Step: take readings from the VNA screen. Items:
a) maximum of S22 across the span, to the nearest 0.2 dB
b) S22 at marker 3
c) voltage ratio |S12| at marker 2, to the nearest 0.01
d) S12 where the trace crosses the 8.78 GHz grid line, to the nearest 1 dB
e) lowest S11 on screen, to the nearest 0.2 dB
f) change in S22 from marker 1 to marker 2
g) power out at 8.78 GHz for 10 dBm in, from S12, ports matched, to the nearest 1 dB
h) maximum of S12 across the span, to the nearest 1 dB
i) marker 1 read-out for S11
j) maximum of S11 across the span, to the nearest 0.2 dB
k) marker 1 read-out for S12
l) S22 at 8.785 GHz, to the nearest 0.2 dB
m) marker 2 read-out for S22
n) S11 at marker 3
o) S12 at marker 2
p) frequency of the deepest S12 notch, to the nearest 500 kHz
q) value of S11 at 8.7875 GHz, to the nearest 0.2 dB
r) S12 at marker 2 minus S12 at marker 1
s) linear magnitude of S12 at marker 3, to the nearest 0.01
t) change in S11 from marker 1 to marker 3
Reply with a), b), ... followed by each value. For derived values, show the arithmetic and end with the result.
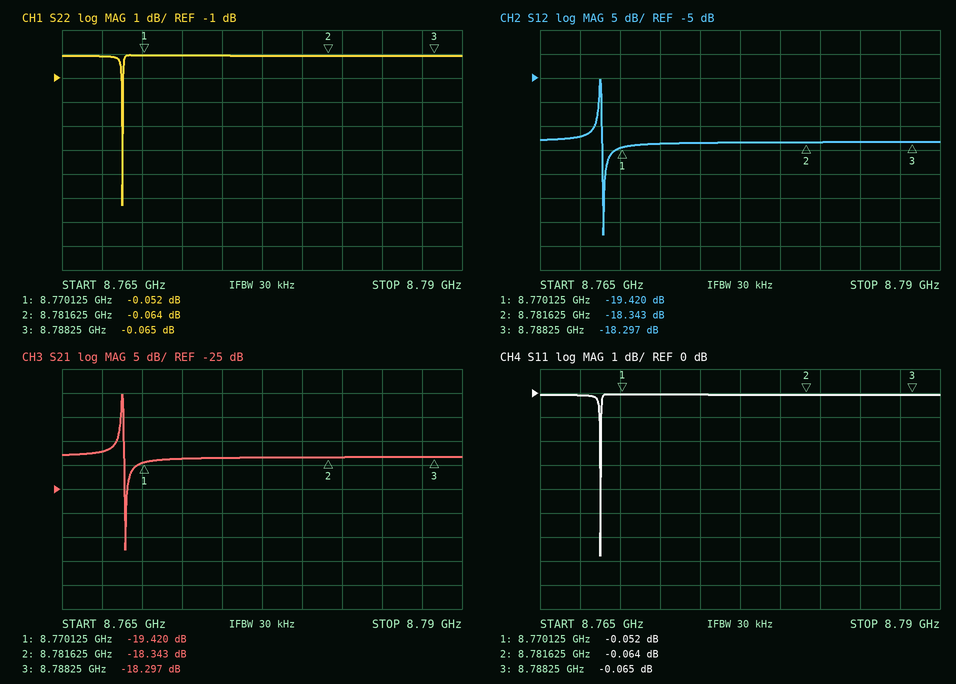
a) 0.0 dB
b) -0.065 dB
c) 10^(-18.343/20) ≈ 0.12
d) -18 dB
e) -6.8 dB
f) -0.064 − (-0.052) = -0.012 dB
g) 10 dBm + (-18 dB) = -8 dBm
h) -5 dB
i) -0.052 dB
j) 0.0 dB
k) -19.420 dB
l) 0.0 dB
m) -0.064 dB
n) -0.065 dB
o) -18.343 dB
p) 8.7690 GHz
q) 0.0 dB
r) -18.343 − (-19.42) = 1.077 dB
s) 10^(-18.297/20) ≈ 0.12
t) -0.065 − (-0.052) = -0.013 dB
